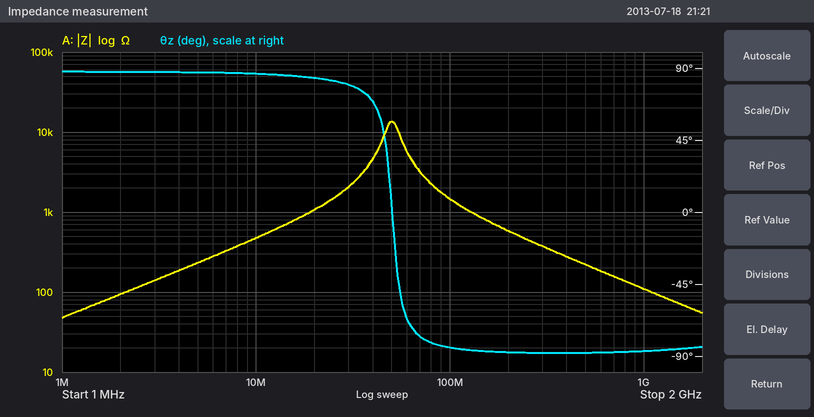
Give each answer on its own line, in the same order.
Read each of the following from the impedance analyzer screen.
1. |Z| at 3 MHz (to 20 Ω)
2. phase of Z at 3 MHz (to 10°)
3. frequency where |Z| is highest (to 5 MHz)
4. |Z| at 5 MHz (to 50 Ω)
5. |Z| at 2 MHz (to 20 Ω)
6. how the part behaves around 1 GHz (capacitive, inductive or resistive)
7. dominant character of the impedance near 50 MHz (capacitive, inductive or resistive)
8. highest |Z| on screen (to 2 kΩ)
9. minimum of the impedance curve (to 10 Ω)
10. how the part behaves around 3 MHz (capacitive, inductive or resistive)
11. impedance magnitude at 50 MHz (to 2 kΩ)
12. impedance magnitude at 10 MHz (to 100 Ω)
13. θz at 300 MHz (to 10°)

140 Ω
90°
50 MHz
250 Ω
100 Ω
capacitive
resistive
14 kΩ
50 Ω
inductive
14 kΩ
500 Ω
-90°
